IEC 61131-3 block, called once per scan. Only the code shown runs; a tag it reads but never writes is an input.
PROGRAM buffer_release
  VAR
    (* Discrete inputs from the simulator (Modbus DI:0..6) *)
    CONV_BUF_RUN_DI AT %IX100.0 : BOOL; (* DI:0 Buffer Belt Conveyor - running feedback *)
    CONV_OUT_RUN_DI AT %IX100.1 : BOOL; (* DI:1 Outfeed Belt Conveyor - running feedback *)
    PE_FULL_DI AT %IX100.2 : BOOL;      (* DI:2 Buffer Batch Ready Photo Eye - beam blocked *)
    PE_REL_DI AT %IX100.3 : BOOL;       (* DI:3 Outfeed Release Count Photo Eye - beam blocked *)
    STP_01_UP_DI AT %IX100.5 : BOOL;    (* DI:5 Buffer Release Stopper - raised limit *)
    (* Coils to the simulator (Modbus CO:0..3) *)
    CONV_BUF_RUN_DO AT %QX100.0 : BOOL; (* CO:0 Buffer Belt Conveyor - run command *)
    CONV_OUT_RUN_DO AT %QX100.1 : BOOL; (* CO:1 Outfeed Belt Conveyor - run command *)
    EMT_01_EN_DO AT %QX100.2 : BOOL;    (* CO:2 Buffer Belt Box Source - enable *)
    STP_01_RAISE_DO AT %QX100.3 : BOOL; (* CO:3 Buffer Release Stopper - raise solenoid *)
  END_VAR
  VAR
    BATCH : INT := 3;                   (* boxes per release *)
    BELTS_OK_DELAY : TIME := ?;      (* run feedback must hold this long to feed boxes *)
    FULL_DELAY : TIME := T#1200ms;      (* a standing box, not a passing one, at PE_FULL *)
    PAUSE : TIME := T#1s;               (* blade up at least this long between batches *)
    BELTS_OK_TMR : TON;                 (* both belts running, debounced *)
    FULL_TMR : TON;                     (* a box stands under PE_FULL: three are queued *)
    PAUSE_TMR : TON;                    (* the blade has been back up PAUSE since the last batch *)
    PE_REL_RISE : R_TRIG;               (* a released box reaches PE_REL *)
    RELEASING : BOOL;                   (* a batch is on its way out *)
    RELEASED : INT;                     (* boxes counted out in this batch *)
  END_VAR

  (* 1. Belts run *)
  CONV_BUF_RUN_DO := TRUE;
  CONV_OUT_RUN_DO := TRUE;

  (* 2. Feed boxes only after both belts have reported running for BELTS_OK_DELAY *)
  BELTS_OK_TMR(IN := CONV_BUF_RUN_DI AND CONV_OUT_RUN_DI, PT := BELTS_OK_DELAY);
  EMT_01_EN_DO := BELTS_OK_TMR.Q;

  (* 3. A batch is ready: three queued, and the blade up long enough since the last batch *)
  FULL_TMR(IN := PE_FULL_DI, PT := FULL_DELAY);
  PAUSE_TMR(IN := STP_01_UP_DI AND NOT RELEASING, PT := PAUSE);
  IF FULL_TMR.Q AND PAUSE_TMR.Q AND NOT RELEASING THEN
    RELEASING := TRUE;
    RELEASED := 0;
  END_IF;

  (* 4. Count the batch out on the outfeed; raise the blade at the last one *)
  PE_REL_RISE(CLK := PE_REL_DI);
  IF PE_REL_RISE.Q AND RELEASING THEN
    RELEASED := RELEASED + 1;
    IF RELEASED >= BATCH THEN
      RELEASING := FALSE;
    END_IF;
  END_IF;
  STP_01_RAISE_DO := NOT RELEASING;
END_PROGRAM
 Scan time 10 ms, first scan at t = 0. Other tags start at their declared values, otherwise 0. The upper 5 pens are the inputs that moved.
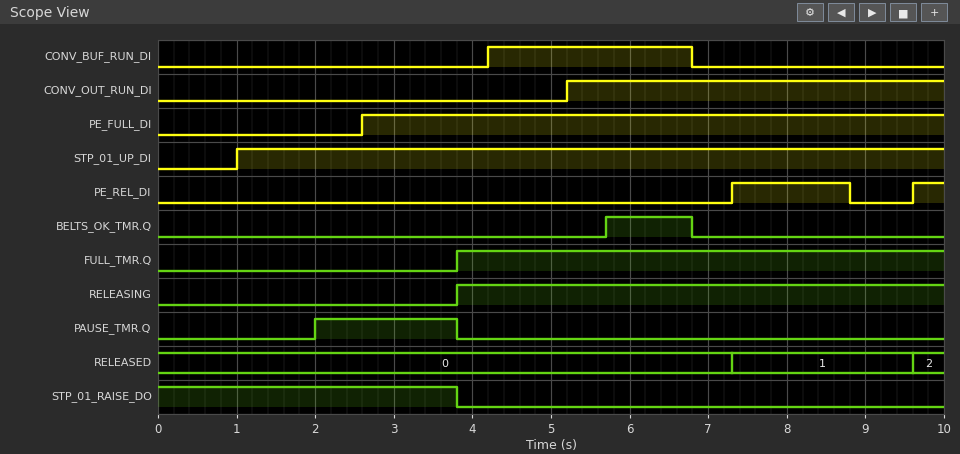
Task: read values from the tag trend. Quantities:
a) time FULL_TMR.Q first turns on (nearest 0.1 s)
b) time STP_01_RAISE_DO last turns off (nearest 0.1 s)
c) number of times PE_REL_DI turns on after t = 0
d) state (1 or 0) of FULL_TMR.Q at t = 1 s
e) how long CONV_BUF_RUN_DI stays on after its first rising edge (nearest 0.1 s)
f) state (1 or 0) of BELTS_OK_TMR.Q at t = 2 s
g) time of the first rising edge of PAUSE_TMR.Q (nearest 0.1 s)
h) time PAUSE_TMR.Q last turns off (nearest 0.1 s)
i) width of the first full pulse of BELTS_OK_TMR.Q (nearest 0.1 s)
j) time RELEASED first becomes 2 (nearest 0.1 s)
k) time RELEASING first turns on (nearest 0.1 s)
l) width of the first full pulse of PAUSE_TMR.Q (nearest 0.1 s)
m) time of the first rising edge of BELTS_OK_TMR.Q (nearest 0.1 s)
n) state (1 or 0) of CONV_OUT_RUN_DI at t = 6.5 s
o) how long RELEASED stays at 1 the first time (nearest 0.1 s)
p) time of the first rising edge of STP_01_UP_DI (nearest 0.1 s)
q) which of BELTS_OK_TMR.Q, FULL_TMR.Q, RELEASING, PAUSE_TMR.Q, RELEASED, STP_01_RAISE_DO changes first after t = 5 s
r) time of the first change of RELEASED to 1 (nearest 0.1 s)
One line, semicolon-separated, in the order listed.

3.8 s; 3.8 s; 2; 0; 2.6 s; 0; 2.0 s; 3.8 s; 1.1 s; 9.6 s; 3.8 s; 1.8 s; 5.7 s; 1; 2.3 s; 1.0 s; BELTS_OK_TMR.Q; 7.3 s
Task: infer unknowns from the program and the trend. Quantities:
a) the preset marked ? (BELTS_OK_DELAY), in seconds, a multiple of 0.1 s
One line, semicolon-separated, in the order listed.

0.5 s
